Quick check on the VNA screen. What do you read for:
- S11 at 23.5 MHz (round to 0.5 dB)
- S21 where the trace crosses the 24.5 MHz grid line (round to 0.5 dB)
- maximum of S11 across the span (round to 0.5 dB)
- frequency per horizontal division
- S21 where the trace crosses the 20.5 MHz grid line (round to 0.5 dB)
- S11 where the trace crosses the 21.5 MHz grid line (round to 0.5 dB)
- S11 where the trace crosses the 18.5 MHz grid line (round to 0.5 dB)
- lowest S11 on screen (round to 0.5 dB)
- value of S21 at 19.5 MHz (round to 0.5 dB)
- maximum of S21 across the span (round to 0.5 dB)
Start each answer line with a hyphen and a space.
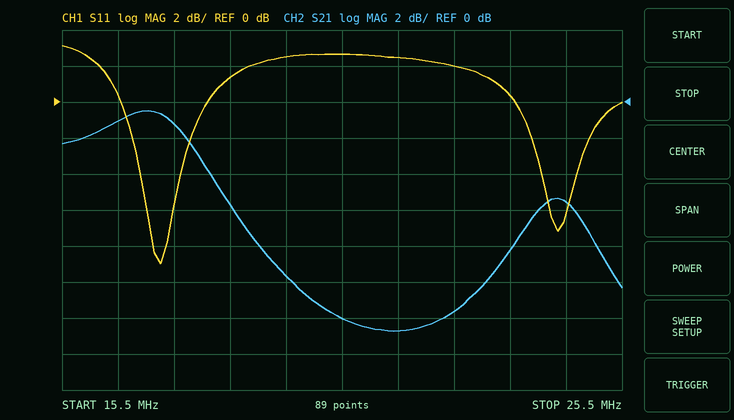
- 0.5 dB
- -5.5 dB
- 3.0 dB
- 1 MHz
- -12.0 dB
- 2.5 dB
- 1.5 dB
- -9.0 dB
- -9.5 dB
- -0.5 dB
